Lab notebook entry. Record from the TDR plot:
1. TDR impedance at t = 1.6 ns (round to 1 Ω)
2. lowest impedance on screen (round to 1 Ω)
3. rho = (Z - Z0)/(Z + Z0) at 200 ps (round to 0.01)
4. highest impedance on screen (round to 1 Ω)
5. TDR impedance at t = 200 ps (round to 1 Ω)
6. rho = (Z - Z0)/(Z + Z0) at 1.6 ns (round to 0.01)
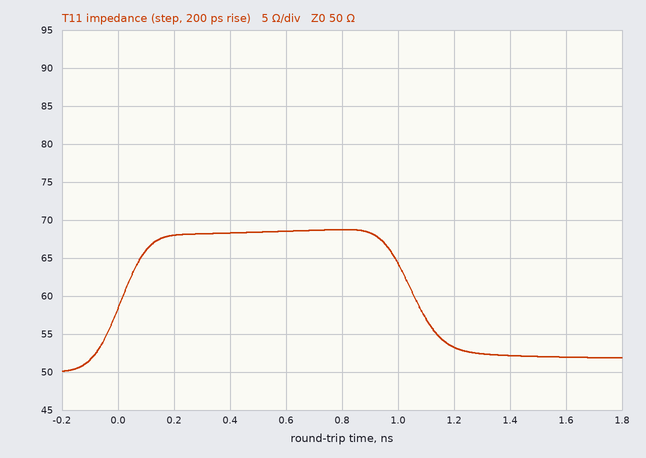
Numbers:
52 Ω
50 Ω
+0.15
69 Ω
68 Ω
+0.02
